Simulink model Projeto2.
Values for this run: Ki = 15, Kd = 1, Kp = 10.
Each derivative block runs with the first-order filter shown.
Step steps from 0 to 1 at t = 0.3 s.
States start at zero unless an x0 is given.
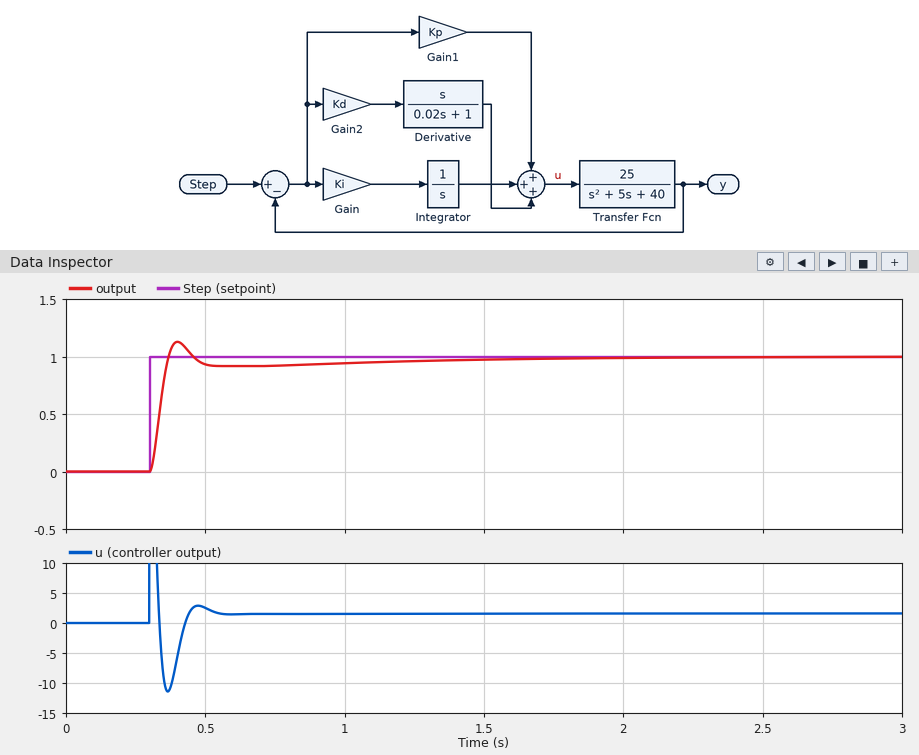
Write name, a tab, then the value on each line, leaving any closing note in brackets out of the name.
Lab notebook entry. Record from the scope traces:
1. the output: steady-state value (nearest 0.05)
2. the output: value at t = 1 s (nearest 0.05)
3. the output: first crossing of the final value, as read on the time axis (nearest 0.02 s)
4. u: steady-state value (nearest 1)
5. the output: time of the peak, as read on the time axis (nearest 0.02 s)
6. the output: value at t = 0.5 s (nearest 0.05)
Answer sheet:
the output: steady-state value	1.00
the output: value at t = 1 s	0.95
the output: first crossing of the final value, as read on the time axis	0.36 s
u: steady-state value	2
the output: time of the peak, as read on the time axis	0.40 s
the output: value at t = 0.5 s	0.95
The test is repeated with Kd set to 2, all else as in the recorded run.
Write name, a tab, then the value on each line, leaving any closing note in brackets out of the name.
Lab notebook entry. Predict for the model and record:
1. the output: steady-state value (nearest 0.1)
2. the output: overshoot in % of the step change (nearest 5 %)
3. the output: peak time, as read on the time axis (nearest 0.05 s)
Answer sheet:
the output: steady-state value	1.0
the output: overshoot in % of the step change	15 %
the output: peak time, as read on the time axis	0.35 s
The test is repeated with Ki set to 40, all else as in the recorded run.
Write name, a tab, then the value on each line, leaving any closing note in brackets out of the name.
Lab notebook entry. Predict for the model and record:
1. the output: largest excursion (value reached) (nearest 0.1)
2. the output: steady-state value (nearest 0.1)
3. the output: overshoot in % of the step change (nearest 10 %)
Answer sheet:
the output: largest excursion (value reached)	1.2
the output: steady-state value	1.0
the output: overshoot in % of the step change	20 %
